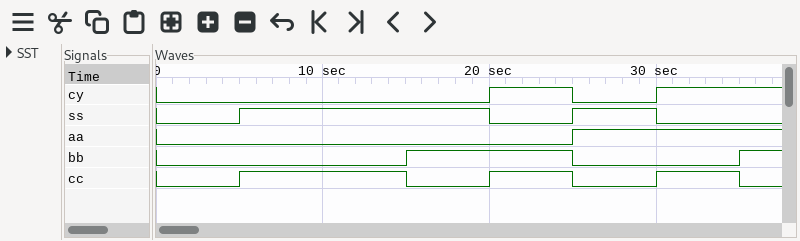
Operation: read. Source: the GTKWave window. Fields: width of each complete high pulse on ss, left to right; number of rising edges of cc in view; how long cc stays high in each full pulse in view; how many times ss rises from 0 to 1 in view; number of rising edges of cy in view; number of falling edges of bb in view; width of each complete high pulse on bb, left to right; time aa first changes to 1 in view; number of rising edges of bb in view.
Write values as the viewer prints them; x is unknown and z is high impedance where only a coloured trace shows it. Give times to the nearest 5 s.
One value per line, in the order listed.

15 s, 5 s
3
10 s, 5 s, 5 s
2
2
1
10 s
25 s
2
